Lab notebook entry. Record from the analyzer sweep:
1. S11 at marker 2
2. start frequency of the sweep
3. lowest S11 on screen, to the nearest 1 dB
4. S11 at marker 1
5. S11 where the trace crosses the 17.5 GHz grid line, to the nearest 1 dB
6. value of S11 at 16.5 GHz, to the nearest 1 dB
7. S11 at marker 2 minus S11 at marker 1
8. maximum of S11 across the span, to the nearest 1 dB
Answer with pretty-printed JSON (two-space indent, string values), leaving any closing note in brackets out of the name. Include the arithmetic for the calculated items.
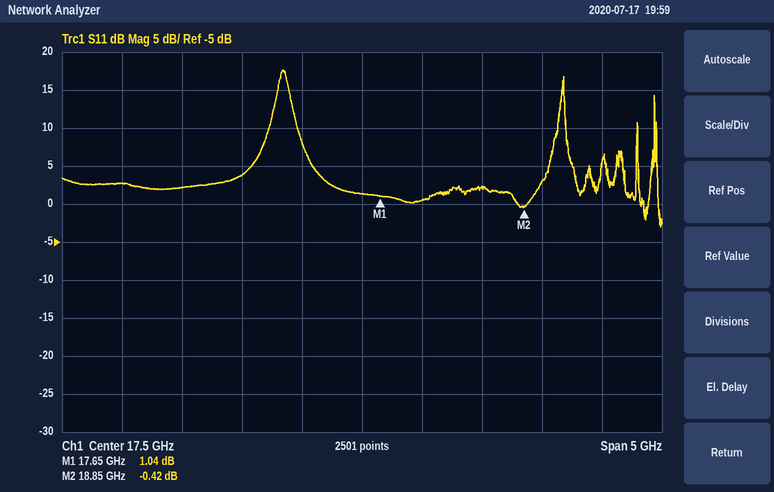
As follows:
{
  "S11 at marker 2": "-0.42 dB",
  "start frequency of the sweep": "15 GHz",
  "lowest S11 on screen, to the nearest 1 dB": "-3 dB",
  "S11 at marker 1": "1.04 dB",
  "S11 where the trace crosses the 17.5 GHz grid line, to the nearest 1 dB": "1 dB",
  "value of S11 at 16.5 GHz, to the nearest 1 dB": "4 dB",
  "S11 at marker 2 minus S11 at marker 1": "-0.42 − (1.04) = -1.46 dB",
  "maximum of S11 across the span, to the nearest 1 dB": "18 dB"
}
